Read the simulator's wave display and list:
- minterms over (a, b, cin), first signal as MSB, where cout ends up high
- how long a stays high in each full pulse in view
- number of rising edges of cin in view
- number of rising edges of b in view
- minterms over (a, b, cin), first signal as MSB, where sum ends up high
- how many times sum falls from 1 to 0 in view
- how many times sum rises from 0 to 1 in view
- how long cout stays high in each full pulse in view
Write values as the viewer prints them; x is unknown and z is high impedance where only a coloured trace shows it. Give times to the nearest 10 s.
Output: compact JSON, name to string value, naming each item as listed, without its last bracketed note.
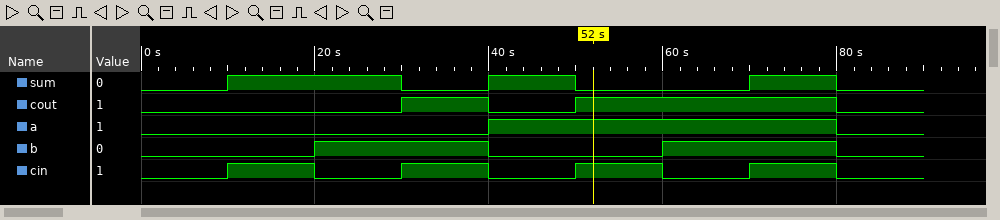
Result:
{"minterms over (a, b, cin), first signal as MSB, where cout ends up high": "3, 5, 6, 7", "how long a stays high in each full pulse in view": "40 s", "number of rising edges of cin in view": "4", "number of rising edges of b in view": "2", "minterms over (a, b, cin), first signal as MSB, where sum ends up high": "1, 2, 4, 7", "how many times sum falls from 1 to 0 in view": "3", "how many times sum rises from 0 to 1 in view": "3", "how long cout stays high in each full pulse in view": "10 s, 30 s"}
